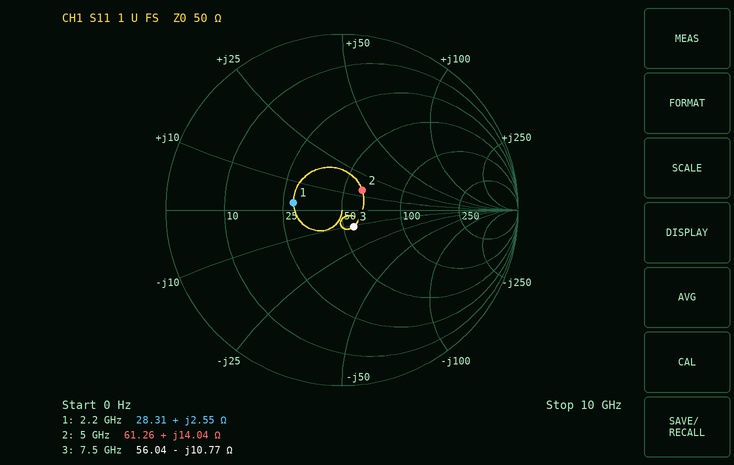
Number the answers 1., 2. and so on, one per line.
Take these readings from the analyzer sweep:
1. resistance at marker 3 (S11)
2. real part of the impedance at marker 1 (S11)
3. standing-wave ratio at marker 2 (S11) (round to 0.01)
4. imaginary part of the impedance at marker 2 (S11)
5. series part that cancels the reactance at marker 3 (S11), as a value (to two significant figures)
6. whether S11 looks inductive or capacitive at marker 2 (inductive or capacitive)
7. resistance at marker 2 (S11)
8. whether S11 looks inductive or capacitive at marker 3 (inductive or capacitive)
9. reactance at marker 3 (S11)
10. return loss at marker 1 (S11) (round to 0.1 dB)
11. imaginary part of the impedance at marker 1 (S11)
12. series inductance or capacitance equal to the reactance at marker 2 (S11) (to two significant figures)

1. 56.04 Ω
2. 28.31 Ω
3. 1.38
4. +14.04 Ω
5. 230 pH
6. inductive
7. 61.26 Ω
8. capacitive
9. -10.77 Ω
10. 11.1 dB
11. +2.55 Ω
12. 450 pH
